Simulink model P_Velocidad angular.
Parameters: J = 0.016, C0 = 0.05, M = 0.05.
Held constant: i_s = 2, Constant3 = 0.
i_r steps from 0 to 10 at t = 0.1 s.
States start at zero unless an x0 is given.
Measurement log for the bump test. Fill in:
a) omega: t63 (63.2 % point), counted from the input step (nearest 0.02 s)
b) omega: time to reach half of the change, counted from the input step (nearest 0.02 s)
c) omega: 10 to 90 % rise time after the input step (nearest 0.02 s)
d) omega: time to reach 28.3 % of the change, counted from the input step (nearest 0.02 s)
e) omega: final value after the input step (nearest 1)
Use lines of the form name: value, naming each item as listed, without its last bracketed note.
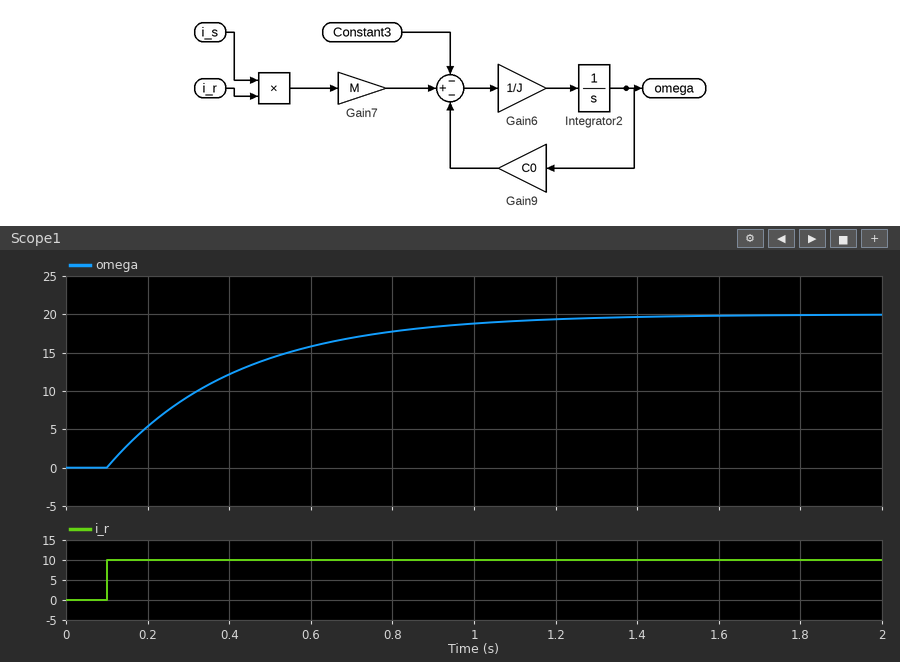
omega: t63 (63.2 % point), counted from the input step: 0.32 s
omega: time to reach half of the change, counted from the input step: 0.22 s
omega: 10 to 90 % rise time after the input step: 0.70 s
omega: time to reach 28.3 % of the change, counted from the input step: 0.10 s
omega: final value after the input step: 20
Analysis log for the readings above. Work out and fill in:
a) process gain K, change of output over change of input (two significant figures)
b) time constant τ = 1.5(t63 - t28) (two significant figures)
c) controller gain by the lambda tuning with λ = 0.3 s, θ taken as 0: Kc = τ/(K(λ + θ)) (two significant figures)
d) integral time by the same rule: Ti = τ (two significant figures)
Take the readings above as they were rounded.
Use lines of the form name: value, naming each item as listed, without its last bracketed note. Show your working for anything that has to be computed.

process gain K, change of output over change of input: (20 - 0) / 10 = 2.0
time constant τ = 1.5(t63 - t28): 1.5 × (0.32 - 0.1) = 0.33 s
controller gain by the lambda tuning with λ = 0.3 s, θ taken as 0: Kc = τ/(K(λ + θ)): 0.33 / (2 × (0.3 + 0)) = 0.55
integral time by the same rule: Ti = τ: 0.33 s
